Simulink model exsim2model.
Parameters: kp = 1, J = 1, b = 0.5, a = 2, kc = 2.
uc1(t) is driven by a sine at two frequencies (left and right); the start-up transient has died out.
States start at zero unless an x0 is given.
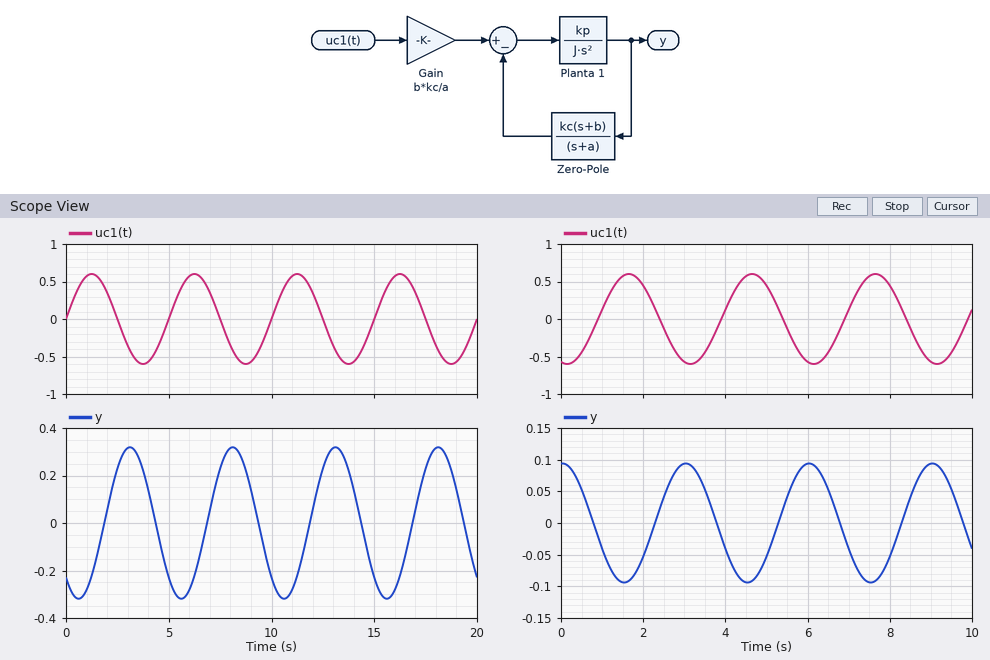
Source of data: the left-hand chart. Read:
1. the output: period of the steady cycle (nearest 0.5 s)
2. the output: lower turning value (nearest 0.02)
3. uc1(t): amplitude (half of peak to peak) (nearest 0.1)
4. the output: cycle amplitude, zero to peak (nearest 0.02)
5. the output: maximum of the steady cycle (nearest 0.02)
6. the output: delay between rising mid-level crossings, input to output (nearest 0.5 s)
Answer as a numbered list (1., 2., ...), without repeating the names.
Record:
1. 5.0 s
2. -0.32
3. 0.6
4. 0.32
5. 0.32
6. 2.0 s
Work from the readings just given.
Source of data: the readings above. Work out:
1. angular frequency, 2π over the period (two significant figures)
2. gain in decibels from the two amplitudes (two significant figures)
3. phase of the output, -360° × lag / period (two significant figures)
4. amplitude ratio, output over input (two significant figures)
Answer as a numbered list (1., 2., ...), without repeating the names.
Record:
1. 1.3 rad/s
2. -5.5 dB
3. -140°
4. 0.53
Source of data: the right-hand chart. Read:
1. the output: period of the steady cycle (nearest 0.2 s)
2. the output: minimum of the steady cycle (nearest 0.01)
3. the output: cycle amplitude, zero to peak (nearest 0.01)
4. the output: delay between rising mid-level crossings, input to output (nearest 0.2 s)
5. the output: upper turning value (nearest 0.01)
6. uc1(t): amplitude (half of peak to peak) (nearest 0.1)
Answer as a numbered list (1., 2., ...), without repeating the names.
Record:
1. 3.0 s
2. -0.09
3. 0.09
4. 1.4 s
5. 0.09
6. 0.6
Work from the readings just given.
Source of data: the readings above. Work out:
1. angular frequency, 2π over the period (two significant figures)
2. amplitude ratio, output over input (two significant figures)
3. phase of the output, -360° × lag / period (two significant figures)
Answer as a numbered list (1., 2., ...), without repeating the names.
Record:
1. 2.1 rad/s
2. 0.15
3. -170°
